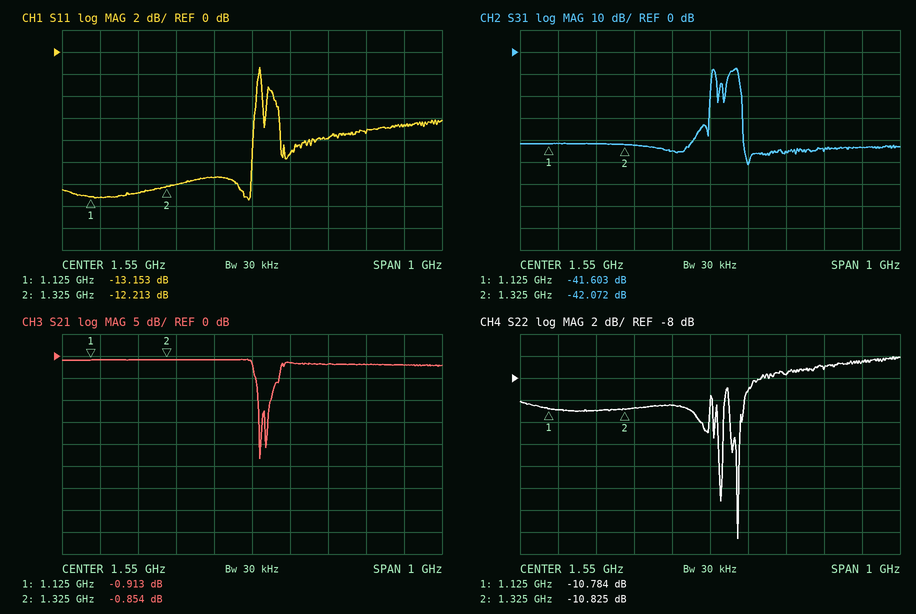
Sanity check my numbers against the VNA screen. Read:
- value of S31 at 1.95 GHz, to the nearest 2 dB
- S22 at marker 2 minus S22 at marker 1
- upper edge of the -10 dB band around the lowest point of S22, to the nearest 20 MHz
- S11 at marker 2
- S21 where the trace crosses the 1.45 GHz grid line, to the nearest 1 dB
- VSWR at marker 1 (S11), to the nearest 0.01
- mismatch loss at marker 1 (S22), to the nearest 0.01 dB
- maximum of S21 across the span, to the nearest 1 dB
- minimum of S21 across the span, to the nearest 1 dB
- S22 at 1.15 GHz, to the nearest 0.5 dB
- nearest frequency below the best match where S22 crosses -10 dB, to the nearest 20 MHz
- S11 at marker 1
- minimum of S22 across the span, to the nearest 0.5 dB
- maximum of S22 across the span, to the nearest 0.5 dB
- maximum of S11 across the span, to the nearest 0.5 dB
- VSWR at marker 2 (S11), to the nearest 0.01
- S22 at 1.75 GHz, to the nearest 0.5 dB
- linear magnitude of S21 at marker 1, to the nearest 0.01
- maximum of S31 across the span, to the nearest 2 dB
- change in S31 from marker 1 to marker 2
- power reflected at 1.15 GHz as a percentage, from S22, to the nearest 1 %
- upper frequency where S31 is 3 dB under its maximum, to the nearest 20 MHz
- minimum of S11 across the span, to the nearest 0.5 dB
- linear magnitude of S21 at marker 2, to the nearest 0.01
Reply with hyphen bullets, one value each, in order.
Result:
- -44 dB
- -0.041 dB
- 1.64 GHz
- -12.213 dB
- -1 dB
- 1.56
- 0.38 dB
- -1 dB
- -23 dB
- -11.0 dB
- 1.60 GHz
- -13.153 dB
- -22.5 dB
- -6.0 dB
- -1.5 dB
- 1.65
- -7.5 dB
- 0.90
- -8 dB
- -0.469 dB
- 8 %
- 1.62 GHz
- -13.5 dB
- 0.91
